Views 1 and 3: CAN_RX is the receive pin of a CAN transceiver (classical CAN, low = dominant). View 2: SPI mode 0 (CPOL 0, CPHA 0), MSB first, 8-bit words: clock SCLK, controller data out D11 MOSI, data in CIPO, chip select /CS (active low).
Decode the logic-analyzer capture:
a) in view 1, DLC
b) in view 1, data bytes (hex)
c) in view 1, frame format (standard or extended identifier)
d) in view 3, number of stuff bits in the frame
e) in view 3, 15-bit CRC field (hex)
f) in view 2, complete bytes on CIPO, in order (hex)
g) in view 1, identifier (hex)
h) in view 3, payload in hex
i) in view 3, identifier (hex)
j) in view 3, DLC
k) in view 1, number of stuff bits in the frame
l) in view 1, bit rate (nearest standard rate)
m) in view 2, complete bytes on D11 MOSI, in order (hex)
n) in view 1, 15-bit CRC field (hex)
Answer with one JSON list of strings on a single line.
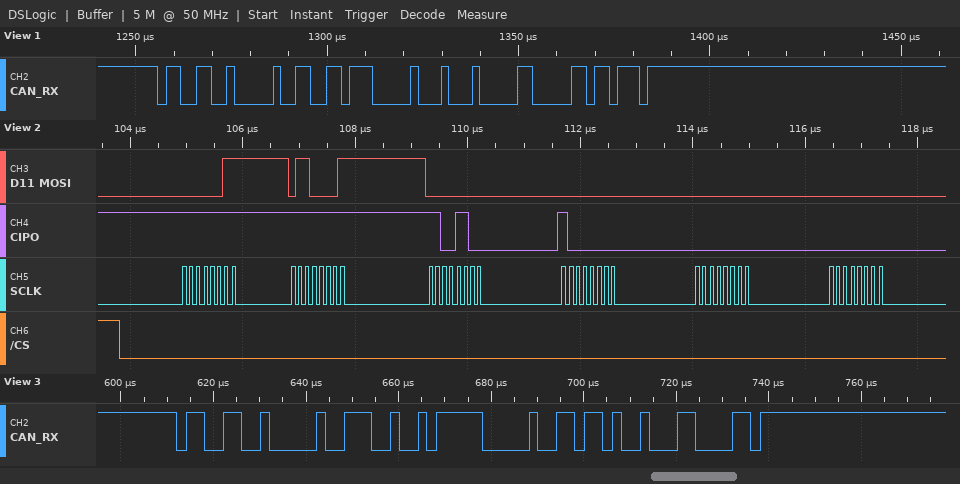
["3", "37 00 88", "standard", "3", "0x2461", "0xFF 0xFF 0xCC 0x80 0x00 0x00", "0x664", "92 F8 1B", "0x664", "3", "4", "500 kbit/s", "0x03 0x61 0x00 0x00 0x00 0x00", "0x105B"]
